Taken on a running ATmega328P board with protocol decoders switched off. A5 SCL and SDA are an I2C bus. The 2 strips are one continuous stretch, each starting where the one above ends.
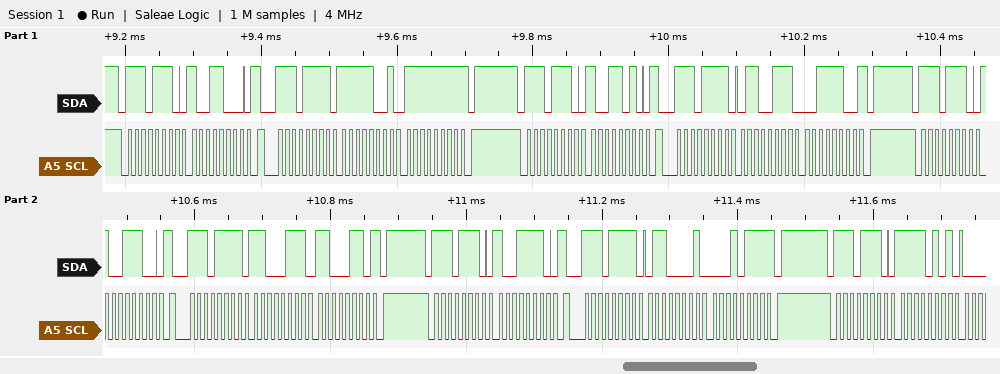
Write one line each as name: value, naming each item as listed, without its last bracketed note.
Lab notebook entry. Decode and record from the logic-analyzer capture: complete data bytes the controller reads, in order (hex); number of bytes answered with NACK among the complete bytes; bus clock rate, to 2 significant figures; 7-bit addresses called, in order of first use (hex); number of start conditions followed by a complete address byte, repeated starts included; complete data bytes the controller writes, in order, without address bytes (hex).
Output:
complete data bytes the controller reads, in order: F9 FF 67 3C C7 C6 61 17
number of bytes answered with NACK among the complete bytes: 4
bus clock rate, to 2 significant figures: 100 kHz
7-bit addresses called, in order of first use: 0x77
number of start conditions followed by a complete address byte, repeated starts included: 9
complete data bytes the controller writes, in order, without address bytes: 98 9A 9C 9E F5
